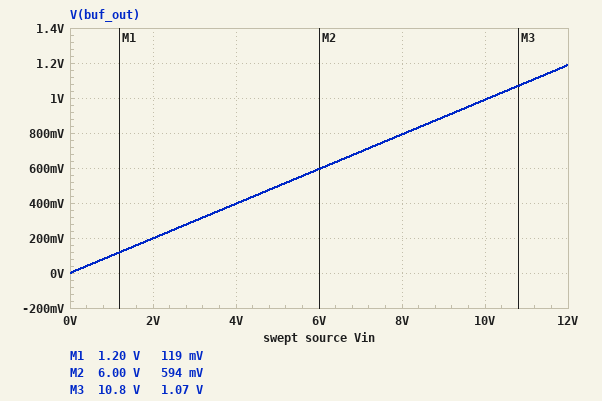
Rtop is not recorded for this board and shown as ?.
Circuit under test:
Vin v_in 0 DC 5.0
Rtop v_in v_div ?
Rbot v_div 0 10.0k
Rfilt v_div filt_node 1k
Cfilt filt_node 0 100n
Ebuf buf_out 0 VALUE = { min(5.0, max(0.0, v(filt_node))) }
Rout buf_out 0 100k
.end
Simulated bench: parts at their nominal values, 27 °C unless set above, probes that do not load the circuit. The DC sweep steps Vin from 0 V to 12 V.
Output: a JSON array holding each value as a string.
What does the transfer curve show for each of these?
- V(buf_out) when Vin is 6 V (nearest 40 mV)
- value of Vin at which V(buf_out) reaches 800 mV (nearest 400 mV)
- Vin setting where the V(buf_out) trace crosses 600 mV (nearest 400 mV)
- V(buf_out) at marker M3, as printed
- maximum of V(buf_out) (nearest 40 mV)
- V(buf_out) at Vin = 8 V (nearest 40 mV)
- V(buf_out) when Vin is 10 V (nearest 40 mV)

["600 mV", "8.0 V", "6.0 V", "1.07 V", "1.20 V", "800 mV", "1.00 V"]
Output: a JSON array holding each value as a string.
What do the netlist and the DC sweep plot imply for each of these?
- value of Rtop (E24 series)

["91 kΩ"]
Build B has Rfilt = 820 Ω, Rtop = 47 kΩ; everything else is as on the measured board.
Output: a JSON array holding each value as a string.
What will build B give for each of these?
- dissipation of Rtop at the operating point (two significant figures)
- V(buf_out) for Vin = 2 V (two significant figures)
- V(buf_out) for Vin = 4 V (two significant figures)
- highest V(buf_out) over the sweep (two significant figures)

["360 µW", "350 mV", "700 mV", "2.1 V"]
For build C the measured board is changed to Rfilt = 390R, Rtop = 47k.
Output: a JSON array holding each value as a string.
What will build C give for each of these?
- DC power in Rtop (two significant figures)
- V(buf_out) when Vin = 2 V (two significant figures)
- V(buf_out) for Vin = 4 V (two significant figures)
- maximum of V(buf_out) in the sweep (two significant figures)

["360 µW", "350 mV", "700 mV", "2.1 V"]
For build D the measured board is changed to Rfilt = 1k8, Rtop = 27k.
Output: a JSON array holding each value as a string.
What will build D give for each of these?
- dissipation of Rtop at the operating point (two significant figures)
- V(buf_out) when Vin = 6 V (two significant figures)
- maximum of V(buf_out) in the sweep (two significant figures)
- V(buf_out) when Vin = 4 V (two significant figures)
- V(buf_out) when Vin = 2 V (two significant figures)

["490 µW", "1.6 V", "3.2 V", "1.1 V", "540 mV"]
